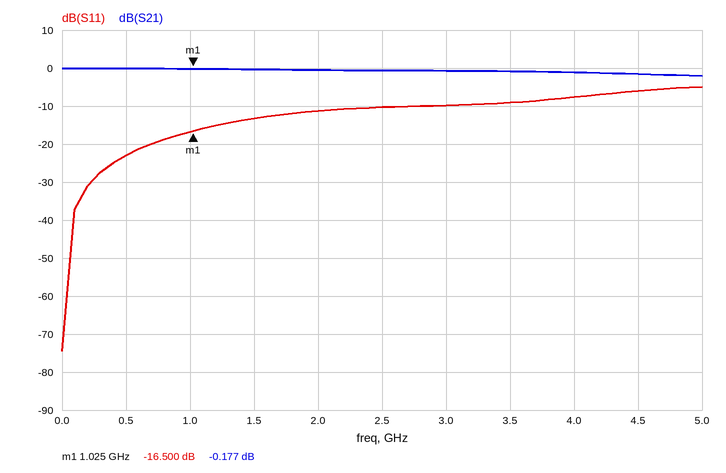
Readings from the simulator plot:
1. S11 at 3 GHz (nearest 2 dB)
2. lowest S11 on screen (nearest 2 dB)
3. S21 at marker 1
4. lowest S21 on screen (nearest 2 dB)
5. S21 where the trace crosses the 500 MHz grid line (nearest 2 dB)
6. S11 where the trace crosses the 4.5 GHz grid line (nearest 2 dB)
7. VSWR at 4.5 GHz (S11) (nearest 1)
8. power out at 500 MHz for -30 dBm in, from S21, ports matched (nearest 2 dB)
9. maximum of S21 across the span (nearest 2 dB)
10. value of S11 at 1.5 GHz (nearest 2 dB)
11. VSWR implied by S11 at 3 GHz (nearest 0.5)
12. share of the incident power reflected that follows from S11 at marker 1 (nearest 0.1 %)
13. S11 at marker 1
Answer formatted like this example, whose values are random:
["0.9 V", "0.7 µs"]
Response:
["-10 dB", "-74 dB", "-0.177 dB", "-2 dB", "0 dB", "-6 dB", "3", "-30 dBm", "0 dB", "-14 dB", "2.0", "2.2 %", "-16.500 dB"]
